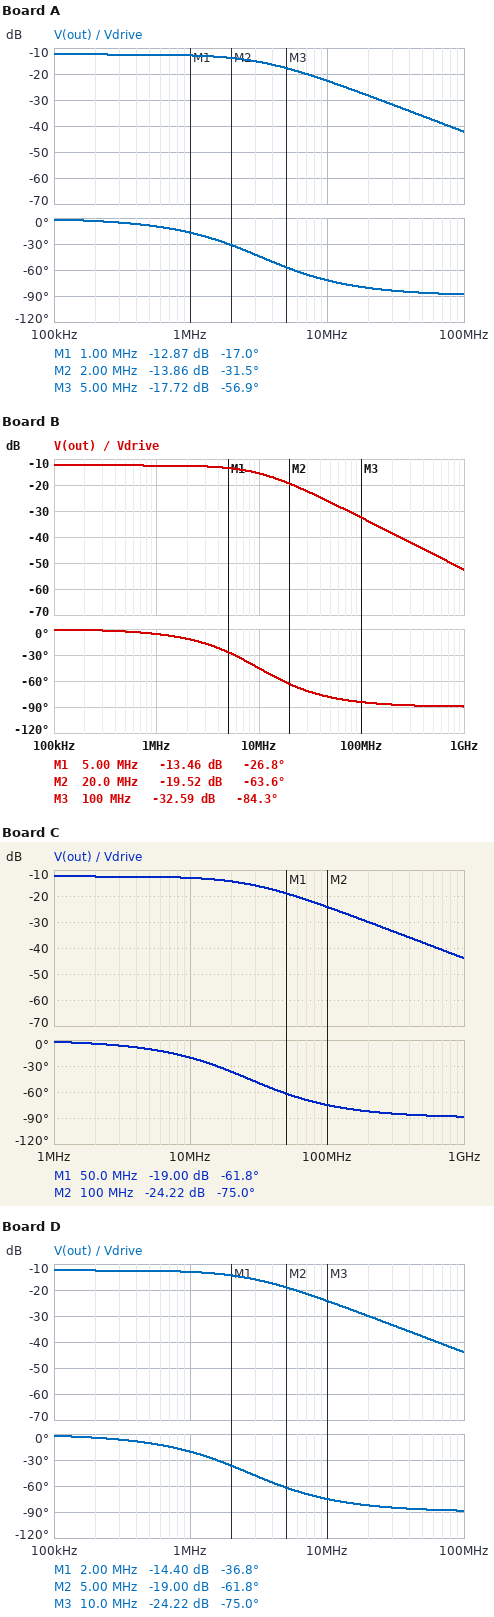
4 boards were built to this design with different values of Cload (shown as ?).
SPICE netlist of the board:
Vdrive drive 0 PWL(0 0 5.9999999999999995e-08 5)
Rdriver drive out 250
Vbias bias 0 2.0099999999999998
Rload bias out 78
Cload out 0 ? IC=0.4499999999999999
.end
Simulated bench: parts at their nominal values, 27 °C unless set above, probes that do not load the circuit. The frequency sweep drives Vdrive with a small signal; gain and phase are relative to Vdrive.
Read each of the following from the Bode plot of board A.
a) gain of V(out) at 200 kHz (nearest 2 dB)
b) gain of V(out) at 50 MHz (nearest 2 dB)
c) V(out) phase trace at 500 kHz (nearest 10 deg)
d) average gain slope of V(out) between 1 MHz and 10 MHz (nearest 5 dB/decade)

-12 dB
-36 dB
-10 deg
-10 dB/decade
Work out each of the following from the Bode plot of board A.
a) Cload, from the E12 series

820 pF
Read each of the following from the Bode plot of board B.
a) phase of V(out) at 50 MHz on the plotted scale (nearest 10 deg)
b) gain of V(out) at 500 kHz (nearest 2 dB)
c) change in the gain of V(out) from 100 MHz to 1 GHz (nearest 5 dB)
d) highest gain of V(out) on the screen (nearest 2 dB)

-80 deg
-12 dB
-20 dB
-12 dB
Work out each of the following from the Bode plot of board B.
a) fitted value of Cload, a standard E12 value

270 pF
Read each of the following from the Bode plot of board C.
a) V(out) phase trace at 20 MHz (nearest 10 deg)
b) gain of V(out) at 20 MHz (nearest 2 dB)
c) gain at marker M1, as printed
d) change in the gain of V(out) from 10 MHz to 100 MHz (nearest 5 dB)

-40 deg
-14 dB
-19.00 dB
-10 dB
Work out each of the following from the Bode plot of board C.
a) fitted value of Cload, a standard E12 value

100 pF
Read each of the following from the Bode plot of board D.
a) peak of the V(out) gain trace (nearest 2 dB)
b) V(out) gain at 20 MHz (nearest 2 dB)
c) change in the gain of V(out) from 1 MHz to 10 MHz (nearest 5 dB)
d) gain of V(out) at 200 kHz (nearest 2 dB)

-12 dB
-30 dB
-10 dB
-12 dB
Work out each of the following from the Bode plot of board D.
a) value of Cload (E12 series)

1 nF
